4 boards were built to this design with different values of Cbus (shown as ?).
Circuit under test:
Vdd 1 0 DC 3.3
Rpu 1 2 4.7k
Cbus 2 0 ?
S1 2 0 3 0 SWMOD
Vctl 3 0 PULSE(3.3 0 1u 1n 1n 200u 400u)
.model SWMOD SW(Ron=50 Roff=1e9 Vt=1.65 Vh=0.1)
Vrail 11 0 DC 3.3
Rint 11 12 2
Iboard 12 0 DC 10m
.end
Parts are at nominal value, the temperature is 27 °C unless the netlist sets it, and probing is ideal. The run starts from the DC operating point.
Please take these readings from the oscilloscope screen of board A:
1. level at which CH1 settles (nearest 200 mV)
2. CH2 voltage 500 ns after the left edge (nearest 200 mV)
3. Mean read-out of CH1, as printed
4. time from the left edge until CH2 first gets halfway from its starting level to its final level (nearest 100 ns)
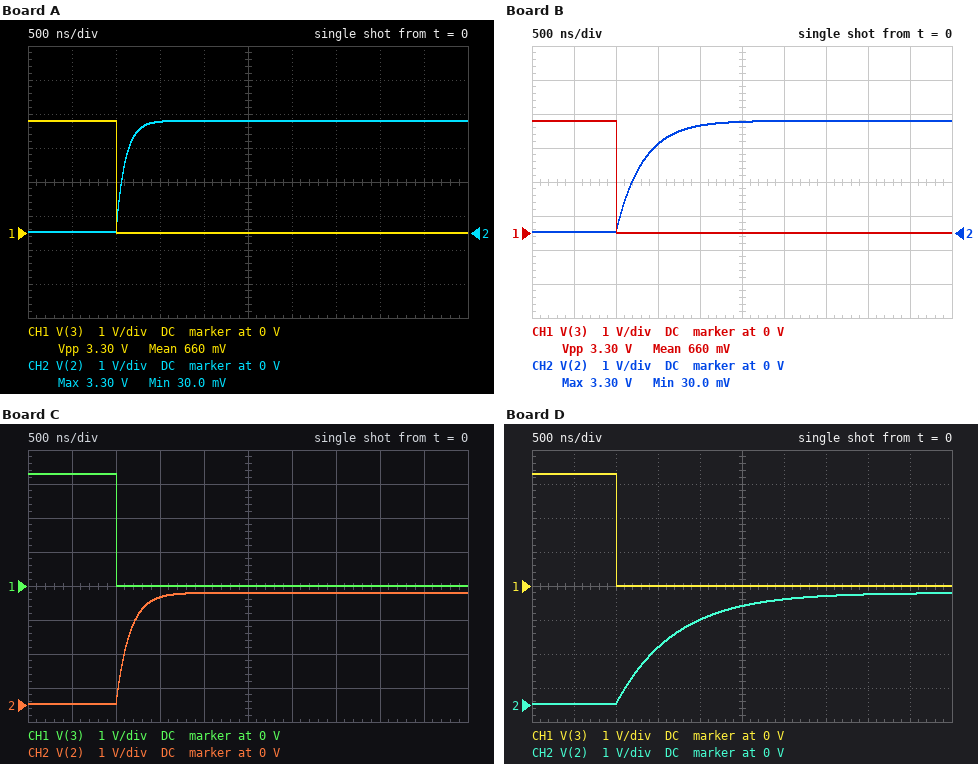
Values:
0 V
0 V
660 mV
1.1 µs
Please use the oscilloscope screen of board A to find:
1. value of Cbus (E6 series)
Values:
22 pF
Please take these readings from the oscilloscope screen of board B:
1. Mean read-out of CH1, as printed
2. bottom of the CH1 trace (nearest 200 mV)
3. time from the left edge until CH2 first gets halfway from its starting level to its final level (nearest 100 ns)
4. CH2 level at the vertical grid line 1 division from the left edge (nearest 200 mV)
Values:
660 mV
0 V
1.2 µs
0 V
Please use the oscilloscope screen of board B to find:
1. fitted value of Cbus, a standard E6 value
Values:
68 pF
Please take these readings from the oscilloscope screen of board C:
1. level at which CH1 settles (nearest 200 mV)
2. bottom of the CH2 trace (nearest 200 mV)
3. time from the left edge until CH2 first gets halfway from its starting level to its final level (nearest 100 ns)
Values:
0 V
0 V
1.1 µs
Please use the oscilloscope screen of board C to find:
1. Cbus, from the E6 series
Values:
33 pF
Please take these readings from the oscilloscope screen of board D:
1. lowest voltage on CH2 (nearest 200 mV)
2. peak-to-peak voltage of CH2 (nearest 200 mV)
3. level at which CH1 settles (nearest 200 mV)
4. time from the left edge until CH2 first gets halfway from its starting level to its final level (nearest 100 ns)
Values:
0 V
3.2 V
0 V
1.5 µs
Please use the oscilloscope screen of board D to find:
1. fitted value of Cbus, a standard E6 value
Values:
150 pF
